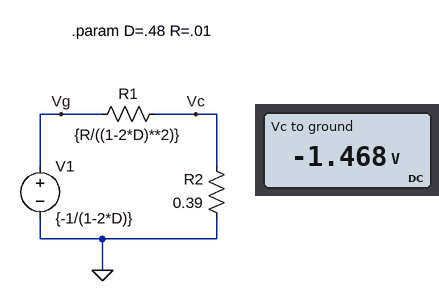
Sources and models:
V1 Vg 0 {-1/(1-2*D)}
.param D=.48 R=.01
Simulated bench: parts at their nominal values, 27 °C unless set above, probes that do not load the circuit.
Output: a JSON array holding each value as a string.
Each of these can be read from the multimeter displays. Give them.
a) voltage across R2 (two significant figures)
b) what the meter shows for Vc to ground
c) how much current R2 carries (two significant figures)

["1.5 V", "-1.468 V", "3.8 A"]
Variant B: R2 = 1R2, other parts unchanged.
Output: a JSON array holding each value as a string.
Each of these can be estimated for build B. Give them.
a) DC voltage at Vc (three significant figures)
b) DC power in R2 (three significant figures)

["-4.03 V", "13.5 W"]
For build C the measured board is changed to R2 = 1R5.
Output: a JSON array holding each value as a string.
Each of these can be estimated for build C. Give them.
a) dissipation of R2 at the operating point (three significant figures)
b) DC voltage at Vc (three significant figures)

["15.6 W", "-4.84 V"]
